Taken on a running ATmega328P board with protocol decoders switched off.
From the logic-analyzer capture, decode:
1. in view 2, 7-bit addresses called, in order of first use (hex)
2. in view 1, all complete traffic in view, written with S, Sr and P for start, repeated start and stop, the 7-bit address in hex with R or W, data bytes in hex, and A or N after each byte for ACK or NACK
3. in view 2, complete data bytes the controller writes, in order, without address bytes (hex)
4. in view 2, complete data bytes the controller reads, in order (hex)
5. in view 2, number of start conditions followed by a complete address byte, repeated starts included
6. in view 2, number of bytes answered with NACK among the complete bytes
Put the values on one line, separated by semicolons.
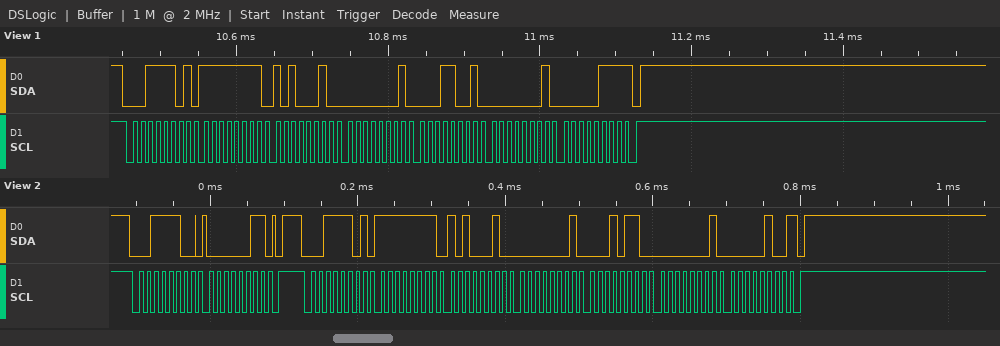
0x1E; S 1ER A FF A A2 A 01 A 19 A 01 A 07 N P; 03; FF A2 01 16 01 04; 2; 1
